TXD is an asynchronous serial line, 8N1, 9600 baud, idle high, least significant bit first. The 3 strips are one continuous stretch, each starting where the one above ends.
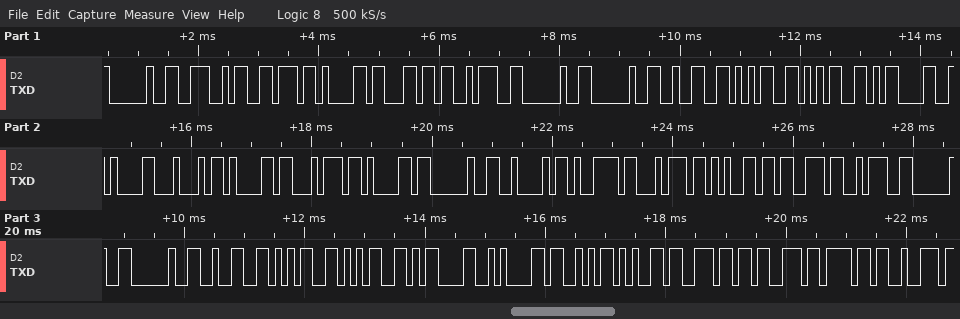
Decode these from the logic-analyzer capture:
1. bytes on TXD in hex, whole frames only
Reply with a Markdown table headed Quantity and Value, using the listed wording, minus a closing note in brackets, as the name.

| Quantity | Value |
|---|---|
| bytes on TXD in hex, whole frames only | 20 4E 76 61 6C 3A 20 20 32 35 35 0D 0A 44 61 74 61 20 42 79 74 65 73 3A 20 20 32 35 35 0D 0A 53 65 6E 73 6F 72 |
